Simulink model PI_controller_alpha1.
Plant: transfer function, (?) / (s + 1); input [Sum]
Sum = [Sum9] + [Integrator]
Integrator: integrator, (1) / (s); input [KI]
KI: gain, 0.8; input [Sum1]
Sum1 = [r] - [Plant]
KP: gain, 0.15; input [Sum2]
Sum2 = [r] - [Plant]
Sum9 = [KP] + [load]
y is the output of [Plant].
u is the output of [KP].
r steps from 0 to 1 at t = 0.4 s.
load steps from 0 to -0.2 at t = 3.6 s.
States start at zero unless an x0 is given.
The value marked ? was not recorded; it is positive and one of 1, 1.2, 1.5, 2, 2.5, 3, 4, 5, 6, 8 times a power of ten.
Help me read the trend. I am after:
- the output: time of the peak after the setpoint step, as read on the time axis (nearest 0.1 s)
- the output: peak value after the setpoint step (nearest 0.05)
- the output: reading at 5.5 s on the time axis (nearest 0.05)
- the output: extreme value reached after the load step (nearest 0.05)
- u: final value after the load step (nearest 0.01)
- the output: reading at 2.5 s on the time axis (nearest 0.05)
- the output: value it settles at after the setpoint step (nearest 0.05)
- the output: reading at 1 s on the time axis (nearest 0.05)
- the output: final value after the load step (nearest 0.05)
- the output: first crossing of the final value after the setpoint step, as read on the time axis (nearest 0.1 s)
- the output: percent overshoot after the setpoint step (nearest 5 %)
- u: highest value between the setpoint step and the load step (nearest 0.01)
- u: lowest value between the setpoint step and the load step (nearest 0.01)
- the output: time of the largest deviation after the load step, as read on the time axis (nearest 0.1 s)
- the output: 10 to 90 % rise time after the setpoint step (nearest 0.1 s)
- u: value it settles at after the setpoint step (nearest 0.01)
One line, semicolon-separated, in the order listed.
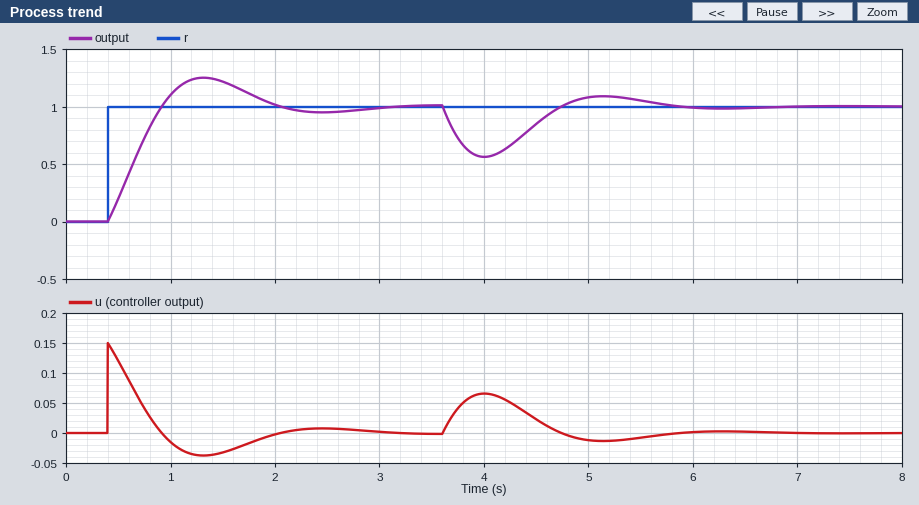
1.3 s; 1.25; 1.05; 0.55; 0.00; 0.95; 1.00; 1.10; 1.00; 0.9 s; 25 %; 0.15; -0.04; 4.0 s; 0.4 s; 0.00
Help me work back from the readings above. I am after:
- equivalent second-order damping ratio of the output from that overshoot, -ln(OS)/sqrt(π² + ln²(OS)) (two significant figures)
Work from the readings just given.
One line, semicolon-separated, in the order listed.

0.40
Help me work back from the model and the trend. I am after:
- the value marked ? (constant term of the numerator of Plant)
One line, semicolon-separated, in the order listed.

12
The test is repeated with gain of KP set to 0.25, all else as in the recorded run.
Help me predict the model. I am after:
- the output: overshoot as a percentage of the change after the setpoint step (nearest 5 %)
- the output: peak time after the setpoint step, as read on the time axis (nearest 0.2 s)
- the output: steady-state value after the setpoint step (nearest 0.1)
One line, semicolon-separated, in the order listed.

15 %; 1.2 s; 1.0
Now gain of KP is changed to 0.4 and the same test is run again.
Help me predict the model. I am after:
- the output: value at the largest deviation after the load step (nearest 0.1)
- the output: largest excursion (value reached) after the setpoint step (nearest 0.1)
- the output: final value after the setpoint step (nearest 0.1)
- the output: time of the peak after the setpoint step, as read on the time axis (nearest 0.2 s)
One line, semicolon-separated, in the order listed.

0.7; 1.1; 1.0; 1.2 s
